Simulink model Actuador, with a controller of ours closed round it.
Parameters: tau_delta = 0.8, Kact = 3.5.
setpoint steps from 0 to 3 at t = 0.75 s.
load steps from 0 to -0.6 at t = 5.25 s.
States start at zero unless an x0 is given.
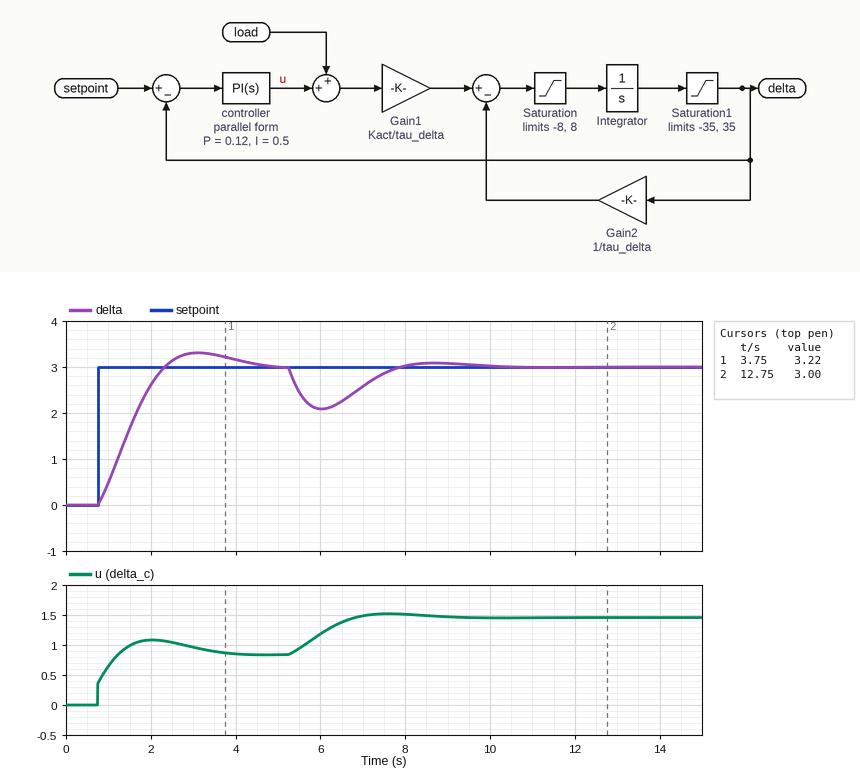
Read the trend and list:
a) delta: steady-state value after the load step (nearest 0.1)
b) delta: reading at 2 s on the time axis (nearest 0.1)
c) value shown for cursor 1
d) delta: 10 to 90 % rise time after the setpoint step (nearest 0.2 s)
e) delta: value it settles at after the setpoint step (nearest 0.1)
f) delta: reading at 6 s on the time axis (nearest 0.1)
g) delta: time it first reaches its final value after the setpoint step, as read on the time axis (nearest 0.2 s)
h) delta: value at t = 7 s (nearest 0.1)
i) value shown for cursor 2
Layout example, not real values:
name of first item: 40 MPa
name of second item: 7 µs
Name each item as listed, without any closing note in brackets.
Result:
delta: steady-state value after the load step: 3.0
delta: reading at 2 s on the time axis: 2.6
value shown for cursor 1: 3.22
delta: 10 to 90 % rise time after the setpoint step: 1.2 s
delta: value it settles at after the setpoint step: 3.0
delta: reading at 6 s on the time axis: 2.1
delta: time it first reaches its final value after the setpoint step, as read on the time axis: 2.4 s
delta: value at t = 7 s: 2.6
value shown for cursor 2: 3.00
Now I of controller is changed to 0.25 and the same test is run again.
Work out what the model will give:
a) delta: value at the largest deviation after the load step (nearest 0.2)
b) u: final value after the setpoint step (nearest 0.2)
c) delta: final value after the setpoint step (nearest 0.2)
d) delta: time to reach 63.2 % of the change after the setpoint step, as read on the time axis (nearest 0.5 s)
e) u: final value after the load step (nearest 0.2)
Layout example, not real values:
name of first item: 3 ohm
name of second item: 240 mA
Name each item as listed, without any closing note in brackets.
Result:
delta: value at the largest deviation after the load step: 2.0
u: final value after the setpoint step: 0.8
delta: final value after the setpoint step: 3.0
delta: time to reach 63.2 % of the change after the setpoint step, as read on the time axis: 2.0 s
u: final value after the load step: 1.4
